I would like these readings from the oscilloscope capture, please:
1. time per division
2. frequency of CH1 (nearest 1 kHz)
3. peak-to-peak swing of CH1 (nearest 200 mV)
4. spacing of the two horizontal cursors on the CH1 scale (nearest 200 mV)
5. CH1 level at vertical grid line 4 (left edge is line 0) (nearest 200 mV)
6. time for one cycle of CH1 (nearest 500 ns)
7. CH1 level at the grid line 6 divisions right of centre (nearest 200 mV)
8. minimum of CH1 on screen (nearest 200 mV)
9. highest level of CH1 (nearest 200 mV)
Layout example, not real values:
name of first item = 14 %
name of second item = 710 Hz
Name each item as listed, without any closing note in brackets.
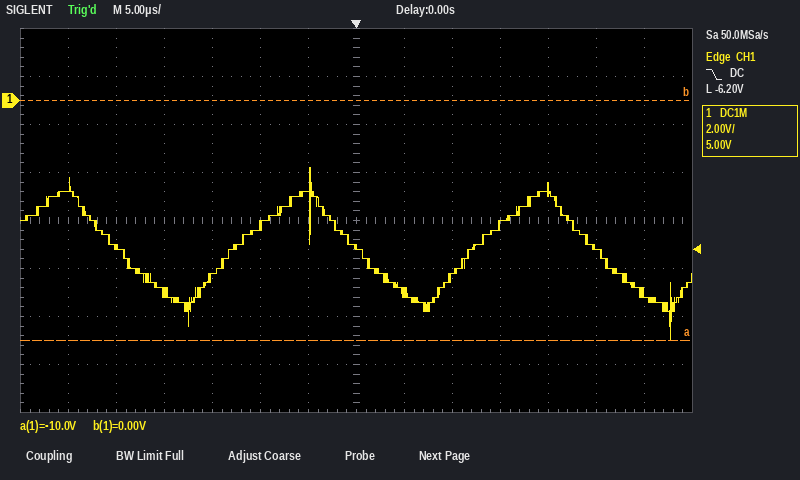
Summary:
time per division = 5 µs
frequency of CH1 = 40 kHz
peak-to-peak swing of CH1 = 7.2 V
spacing of the two horizontal cursors on the CH1 scale = 10.0 V
CH1 level at vertical grid line 4 (left edge is line 0) = -7.4 V
time for one cycle of CH1 = 25.0 µs
CH1 level at the grid line 6 divisions right of centre = -8.0 V
minimum of CH1 on screen = -10.0 V
highest level of CH1 = -2.8 V
